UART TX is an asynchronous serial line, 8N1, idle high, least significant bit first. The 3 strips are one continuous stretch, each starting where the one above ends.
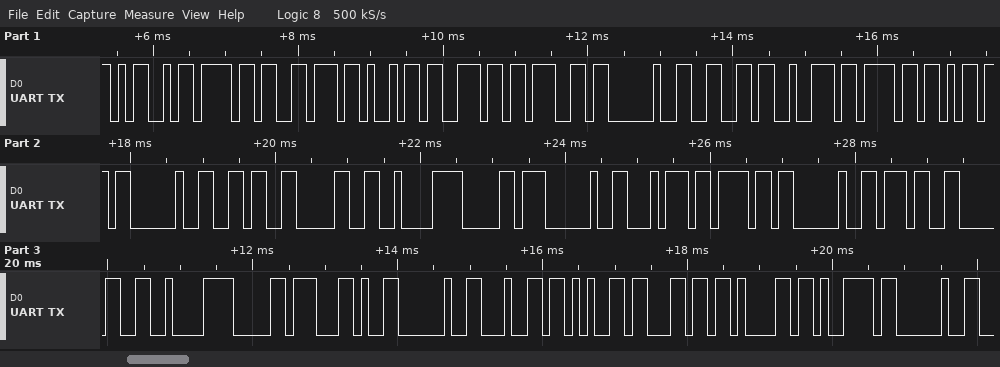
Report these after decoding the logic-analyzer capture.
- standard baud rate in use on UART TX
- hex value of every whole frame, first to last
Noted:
9600 baud
4D 6F 76 69 6E 67 20 66 72 6F 6D 20 36 30 C2 B0 20 74 6F 20 37 30 C2 B0 2C 20 64 65 6C 61 79 20
